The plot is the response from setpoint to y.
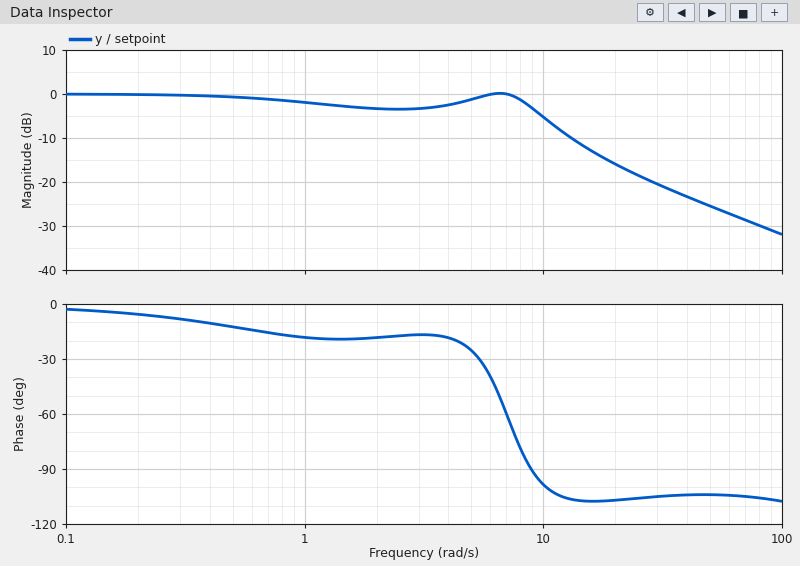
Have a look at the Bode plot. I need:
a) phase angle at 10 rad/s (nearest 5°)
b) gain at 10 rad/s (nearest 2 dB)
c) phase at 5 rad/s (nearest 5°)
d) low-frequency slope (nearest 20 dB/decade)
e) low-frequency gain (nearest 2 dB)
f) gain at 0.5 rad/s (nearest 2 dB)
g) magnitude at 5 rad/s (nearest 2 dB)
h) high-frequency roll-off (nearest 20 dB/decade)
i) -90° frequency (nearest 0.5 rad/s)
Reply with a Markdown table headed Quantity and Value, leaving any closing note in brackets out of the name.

| Quantity | Value |
|---|---|
| phase angle at 10 rad/s | -100° |
| gain at 10 rad/s | -6 dB |
| phase at 5 rad/s | -25° |
| low-frequency slope | 0 dB/decade |
| low-frequency gain | 0 dB |
| gain at 0.5 rad/s | 0 dB |
| magnitude at 5 rad/s | -2 dB |
| high-frequency roll-off | -20 dB/decade |
| -90° frequency | 9.0 rad/s |
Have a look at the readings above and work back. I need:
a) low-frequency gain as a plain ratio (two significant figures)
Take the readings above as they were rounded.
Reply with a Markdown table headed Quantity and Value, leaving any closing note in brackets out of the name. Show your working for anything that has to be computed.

| Quantity | Value |
|---|---|
| low-frequency gain as a plain ratio | 10^(0 / 20) = 1.0 |
